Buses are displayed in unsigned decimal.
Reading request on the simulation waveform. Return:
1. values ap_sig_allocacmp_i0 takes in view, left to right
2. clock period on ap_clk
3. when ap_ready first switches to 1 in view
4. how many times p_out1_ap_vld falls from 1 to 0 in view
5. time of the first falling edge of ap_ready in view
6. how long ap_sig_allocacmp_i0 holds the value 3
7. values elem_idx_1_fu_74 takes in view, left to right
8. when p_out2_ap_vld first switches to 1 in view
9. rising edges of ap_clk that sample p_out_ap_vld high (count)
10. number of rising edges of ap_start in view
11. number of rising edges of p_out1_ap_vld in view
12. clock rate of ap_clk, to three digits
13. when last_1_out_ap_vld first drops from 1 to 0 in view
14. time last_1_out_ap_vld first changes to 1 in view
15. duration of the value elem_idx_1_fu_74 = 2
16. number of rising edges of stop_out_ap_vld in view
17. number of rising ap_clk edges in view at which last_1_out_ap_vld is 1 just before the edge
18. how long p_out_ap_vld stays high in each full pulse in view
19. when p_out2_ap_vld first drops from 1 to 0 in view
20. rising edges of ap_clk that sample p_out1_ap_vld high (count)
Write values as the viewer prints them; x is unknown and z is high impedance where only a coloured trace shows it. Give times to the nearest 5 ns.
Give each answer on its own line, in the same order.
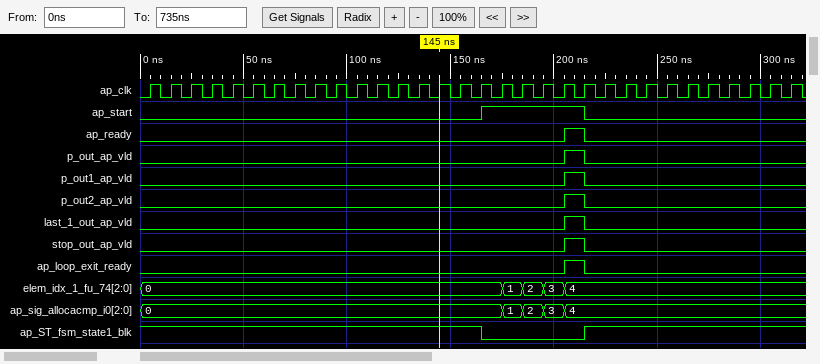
0, 1, 2, 3, 4
10 ns
205 ns
1
215 ns
10 ns
0, 1, 2, 3, 4
205 ns
1
1
1
100 MHz
215 ns
205 ns
10 ns
1
1
10 ns
215 ns
1
